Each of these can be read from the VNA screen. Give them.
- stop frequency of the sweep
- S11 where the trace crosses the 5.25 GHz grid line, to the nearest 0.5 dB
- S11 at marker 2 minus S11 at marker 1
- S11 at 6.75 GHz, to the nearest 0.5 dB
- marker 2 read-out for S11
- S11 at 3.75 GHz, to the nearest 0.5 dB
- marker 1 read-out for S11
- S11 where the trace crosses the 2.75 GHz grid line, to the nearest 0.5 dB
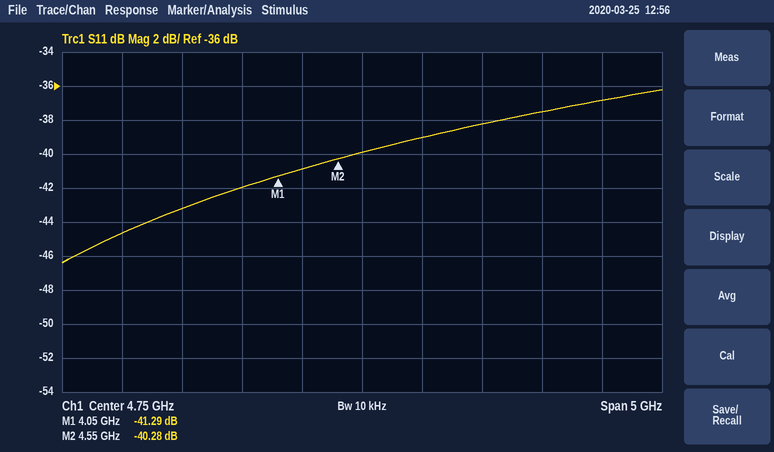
7.25 GHz
-39.0 dB
1.01 dB
-37.0 dB
-40.28 dB
-42.0 dB
-41.29 dB
-44.5 dB
